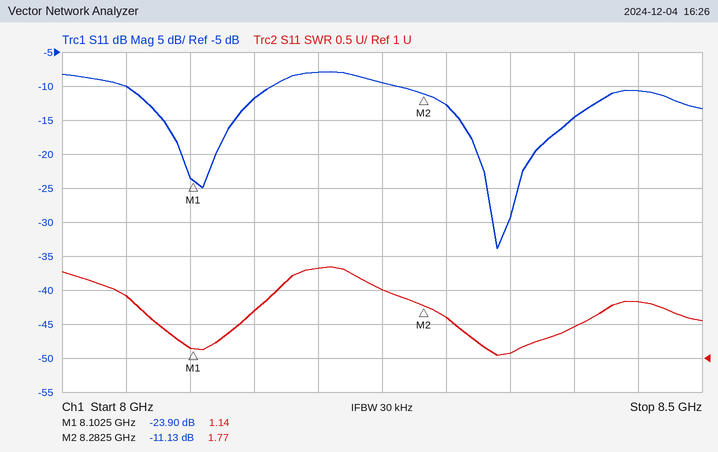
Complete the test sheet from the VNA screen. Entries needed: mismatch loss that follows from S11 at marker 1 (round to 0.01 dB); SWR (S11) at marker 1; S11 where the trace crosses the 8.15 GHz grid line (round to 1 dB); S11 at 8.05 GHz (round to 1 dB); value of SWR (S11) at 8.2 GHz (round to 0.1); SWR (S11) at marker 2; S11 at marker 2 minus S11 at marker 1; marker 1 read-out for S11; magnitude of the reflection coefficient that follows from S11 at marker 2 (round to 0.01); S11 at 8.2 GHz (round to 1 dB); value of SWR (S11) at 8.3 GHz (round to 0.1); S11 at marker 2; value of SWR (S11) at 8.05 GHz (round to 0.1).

0.02 dB
1.14
-12 dB
-10 dB
2.3
1.77
12.77 dB
-23.90 dB
0.28
-8 dB
1.6
-11.13 dB
1.9
